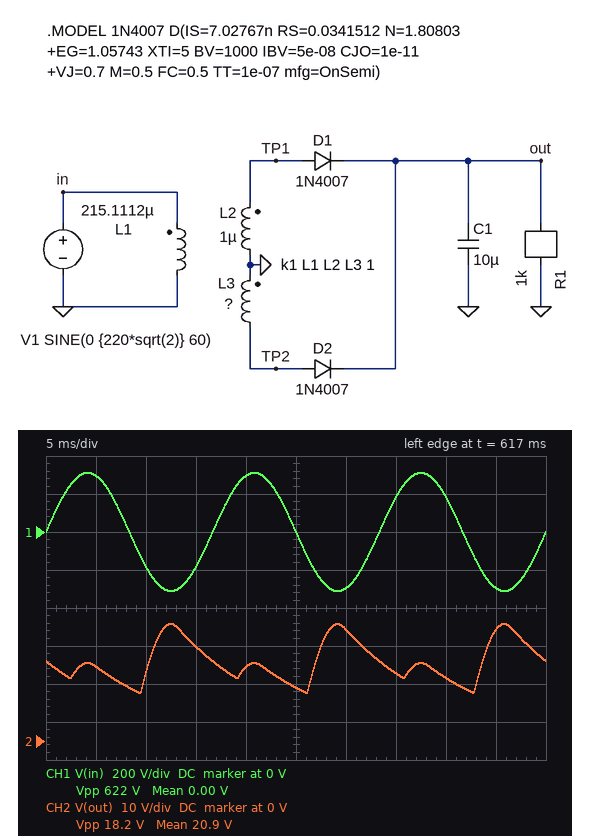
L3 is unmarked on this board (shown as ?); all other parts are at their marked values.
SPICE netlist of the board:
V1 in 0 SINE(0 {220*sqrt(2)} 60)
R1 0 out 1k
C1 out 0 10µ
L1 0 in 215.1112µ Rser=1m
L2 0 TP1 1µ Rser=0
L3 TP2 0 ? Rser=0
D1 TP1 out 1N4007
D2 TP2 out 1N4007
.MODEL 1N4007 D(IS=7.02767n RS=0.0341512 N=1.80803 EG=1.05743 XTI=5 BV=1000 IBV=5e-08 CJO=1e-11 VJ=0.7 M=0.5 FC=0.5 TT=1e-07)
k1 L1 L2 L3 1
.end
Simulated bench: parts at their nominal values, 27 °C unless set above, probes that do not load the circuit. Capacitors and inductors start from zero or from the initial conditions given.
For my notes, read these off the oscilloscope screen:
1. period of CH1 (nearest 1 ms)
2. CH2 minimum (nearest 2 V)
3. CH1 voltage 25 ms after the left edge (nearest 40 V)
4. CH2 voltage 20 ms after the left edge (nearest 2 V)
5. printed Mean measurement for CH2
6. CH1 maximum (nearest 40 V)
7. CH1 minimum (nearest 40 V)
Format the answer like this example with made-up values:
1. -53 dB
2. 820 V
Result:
1. 17 ms
2. 12 V
3. 0 V
4. 20 V
5. 20.9 V
6. 320 V
7. -320 V
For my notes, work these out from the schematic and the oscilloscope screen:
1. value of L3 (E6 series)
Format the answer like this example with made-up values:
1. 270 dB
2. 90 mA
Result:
1. 2.2 µH
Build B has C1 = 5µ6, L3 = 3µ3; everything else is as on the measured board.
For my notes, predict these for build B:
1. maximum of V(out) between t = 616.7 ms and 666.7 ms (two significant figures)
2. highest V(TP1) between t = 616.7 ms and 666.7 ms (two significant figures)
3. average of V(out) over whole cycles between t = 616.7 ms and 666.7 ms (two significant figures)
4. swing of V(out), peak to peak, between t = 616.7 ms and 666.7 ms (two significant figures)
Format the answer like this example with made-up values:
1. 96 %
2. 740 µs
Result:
1. 38 V
2. 21 V
3. 22 V
4. 28 V
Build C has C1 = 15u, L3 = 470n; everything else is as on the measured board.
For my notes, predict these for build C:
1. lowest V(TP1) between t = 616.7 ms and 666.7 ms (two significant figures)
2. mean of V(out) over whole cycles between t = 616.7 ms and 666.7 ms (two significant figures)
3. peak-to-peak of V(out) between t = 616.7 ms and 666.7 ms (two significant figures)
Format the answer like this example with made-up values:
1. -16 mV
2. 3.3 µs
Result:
1. -21 V
2. 15 V
3. 11 V
